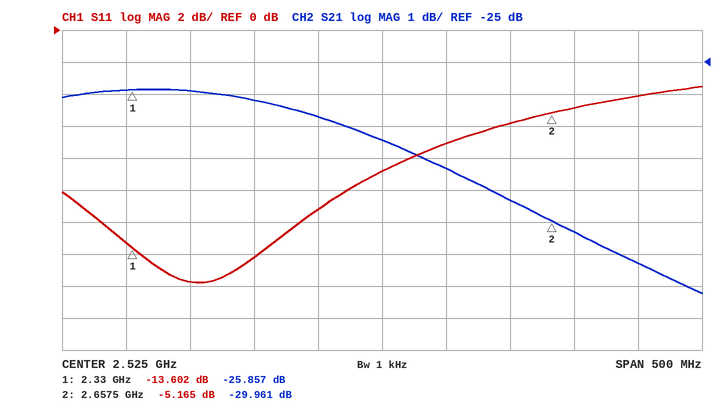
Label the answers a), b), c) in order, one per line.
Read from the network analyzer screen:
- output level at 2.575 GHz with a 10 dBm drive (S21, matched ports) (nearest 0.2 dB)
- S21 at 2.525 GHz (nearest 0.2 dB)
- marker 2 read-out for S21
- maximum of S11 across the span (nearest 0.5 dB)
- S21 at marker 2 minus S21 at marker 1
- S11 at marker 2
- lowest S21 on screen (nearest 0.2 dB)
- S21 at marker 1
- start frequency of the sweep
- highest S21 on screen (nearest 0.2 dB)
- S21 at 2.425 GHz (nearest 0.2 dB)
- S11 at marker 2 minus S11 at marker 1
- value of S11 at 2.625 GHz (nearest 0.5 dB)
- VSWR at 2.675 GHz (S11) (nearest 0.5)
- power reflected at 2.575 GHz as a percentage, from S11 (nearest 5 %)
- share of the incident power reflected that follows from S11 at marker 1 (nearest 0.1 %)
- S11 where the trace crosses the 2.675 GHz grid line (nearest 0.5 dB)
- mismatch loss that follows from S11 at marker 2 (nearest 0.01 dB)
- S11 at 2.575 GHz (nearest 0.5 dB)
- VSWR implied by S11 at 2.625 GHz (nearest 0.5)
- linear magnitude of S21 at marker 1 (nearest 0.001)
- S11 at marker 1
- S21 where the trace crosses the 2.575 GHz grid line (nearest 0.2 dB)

a) -18.4 dBm
b) -27.4 dB
c) -29.961 dB
d) -3.5 dB
e) -4.104 dB
f) -5.165 dB
g) -32.2 dB
h) -25.857 dB
i) 2.275 GHz
j) -25.8 dB
k) -26.2 dB
l) 8.437 dB
m) -6.0 dB
n) 3.5
o) 20 %
p) 4.4 %
q) -5.0 dB
r) 1.58 dB
s) -7.0 dB
t) 3.0
u) 0.051
v) -13.602 dB
w) -28.4 dB
